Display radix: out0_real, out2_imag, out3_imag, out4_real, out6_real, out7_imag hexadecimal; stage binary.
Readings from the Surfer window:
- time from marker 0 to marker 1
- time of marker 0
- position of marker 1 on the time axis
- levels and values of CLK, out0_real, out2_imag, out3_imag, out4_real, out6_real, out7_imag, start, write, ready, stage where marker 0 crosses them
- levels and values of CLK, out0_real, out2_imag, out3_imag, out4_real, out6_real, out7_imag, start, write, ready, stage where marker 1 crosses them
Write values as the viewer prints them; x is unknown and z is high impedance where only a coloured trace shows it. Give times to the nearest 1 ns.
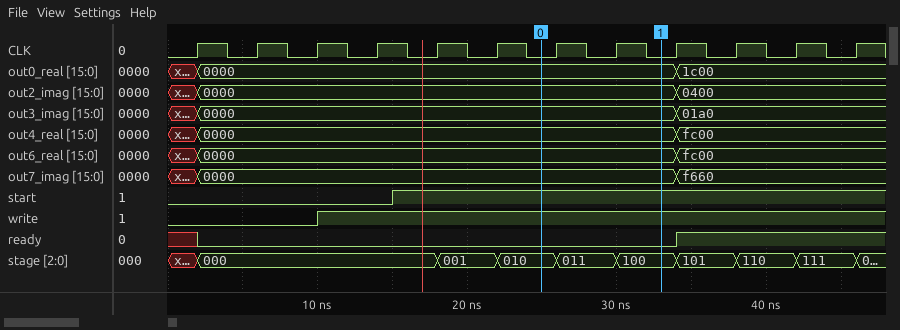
8 ns
25 ns
33 ns
CLK=0, out0_real=0000, out2_imag=0000, out3_imag=0000, out4_real=0000, out6_real=0000, out7_imag=0000, start=1, write=1, ready=0, stage=010
CLK=0, out0_real=0000, out2_imag=0000, out3_imag=0000, out4_real=0000, out6_real=0000, out7_imag=0000, start=1, write=1, ready=0, stage=100
